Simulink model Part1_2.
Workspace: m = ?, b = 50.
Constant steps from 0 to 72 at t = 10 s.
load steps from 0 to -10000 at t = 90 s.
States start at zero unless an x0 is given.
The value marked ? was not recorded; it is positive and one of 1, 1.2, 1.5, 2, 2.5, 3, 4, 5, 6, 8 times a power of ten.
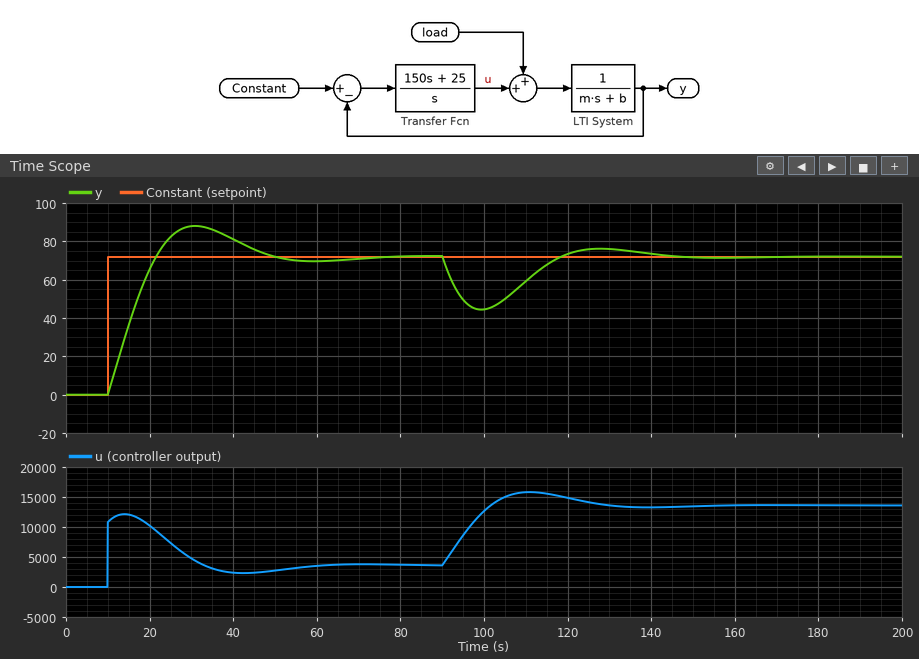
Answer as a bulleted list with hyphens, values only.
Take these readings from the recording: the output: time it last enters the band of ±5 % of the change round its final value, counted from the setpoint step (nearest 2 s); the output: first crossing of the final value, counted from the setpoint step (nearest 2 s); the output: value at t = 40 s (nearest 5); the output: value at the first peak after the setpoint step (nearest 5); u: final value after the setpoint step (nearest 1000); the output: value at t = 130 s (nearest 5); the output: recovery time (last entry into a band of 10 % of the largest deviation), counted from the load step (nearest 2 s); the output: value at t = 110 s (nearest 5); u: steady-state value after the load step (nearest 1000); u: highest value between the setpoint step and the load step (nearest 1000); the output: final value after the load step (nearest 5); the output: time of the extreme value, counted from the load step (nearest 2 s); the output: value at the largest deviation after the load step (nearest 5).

- 36 s
- 12 s
- 80
- 90
- 4000
- 75
- 46 s
- 60
- 14000
- 12000
- 70
- 10 s
- 45
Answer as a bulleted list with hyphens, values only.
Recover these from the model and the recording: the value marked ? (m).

- 1500
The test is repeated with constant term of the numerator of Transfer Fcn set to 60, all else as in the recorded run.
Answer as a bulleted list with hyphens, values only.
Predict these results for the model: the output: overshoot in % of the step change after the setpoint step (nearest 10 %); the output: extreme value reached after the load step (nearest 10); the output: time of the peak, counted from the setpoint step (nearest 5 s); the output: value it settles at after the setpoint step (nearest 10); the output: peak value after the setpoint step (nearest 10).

- 40 %
- 50
- 15 s
- 70
- 100
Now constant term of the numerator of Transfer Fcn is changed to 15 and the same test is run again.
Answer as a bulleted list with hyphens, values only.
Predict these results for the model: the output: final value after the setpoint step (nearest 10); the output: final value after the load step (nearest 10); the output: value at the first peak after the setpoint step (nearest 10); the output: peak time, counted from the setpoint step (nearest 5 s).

- 70
- 70
- 80
- 25 s
